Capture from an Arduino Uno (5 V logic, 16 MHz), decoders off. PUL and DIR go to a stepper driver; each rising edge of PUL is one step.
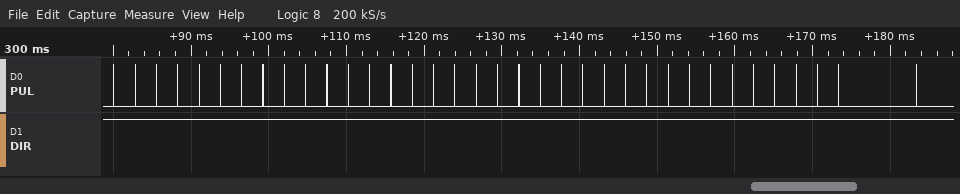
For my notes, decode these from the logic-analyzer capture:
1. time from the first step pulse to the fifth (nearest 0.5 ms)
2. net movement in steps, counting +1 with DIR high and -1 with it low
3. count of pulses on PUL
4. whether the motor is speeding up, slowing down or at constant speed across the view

11.0 ms
+36
36
slowing down
